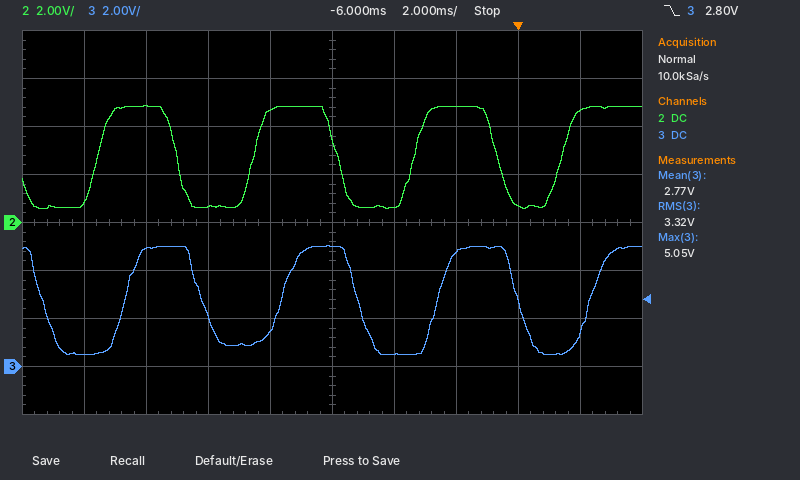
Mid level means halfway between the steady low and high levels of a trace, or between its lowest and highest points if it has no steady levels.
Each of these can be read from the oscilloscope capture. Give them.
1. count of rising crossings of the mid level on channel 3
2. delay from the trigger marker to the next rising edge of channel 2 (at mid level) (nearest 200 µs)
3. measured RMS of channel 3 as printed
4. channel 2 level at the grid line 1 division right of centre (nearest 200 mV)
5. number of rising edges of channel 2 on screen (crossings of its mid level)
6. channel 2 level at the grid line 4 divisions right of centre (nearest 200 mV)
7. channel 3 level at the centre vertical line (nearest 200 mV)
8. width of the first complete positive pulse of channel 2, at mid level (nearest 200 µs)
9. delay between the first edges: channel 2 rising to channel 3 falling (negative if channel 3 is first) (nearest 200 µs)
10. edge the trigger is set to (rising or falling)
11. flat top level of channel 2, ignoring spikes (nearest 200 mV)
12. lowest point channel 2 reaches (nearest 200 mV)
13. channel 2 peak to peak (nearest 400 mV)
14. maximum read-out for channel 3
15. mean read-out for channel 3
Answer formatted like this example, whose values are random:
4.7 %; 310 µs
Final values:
4; 1.4 ms; 3.32 V; 600 mV; 4; 4.6 V; 5.0 V; 2.6 ms; -1.8 ms; falling; 4.8 V; 600 mV; 4.4 V; 5.05 V; 2.77 V
